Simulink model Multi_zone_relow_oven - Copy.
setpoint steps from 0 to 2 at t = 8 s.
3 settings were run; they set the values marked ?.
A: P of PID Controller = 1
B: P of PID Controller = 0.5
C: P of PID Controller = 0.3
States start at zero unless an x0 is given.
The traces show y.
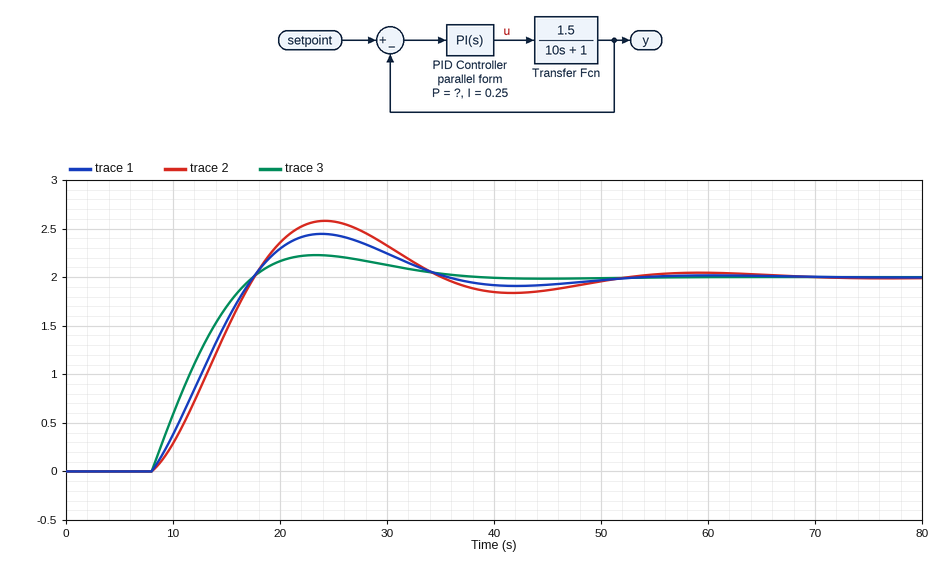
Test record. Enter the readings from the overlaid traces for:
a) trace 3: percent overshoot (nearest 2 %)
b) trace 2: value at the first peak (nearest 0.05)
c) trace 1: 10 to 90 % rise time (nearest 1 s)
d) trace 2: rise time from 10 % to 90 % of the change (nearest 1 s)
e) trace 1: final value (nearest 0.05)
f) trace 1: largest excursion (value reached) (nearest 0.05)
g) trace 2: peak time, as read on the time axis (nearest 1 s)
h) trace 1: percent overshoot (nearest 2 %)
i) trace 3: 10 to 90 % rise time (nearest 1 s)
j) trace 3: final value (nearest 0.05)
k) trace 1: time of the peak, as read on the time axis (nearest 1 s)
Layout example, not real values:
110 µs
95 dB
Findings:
12 %
2.60
7 s
7 s
2.00
2.45
24 s
22 %
7 s
2.00
24 s
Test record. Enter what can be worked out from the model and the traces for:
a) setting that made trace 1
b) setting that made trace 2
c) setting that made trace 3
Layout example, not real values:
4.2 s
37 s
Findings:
B
C
A
